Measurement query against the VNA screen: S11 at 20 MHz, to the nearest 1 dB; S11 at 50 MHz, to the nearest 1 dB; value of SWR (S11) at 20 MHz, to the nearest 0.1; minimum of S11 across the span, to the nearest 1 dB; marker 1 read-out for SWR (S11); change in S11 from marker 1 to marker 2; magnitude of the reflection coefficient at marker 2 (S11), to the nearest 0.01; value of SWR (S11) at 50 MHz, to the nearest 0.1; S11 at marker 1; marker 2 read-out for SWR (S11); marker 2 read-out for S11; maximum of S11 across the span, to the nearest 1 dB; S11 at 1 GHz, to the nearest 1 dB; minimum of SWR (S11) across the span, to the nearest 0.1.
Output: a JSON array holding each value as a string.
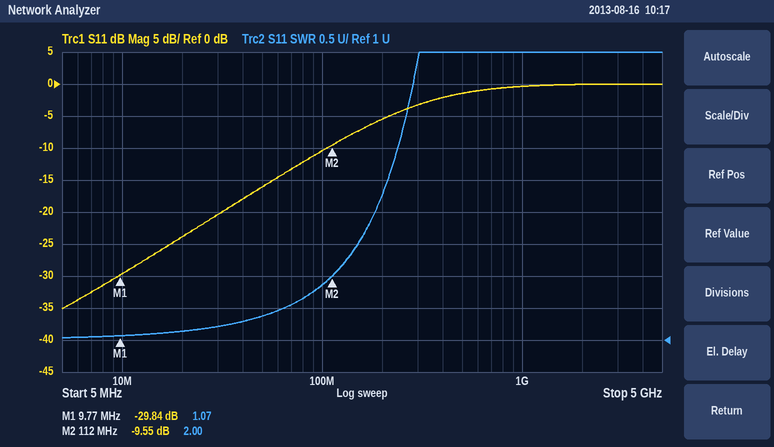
["-24 dB", "-16 dB", "1.1", "-35 dB", "1.07", "20.29 dB", "0.33", "1.4", "-29.84 dB", "2.00", "-9.55 dB", "0 dB", "0 dB", "1.0"]
